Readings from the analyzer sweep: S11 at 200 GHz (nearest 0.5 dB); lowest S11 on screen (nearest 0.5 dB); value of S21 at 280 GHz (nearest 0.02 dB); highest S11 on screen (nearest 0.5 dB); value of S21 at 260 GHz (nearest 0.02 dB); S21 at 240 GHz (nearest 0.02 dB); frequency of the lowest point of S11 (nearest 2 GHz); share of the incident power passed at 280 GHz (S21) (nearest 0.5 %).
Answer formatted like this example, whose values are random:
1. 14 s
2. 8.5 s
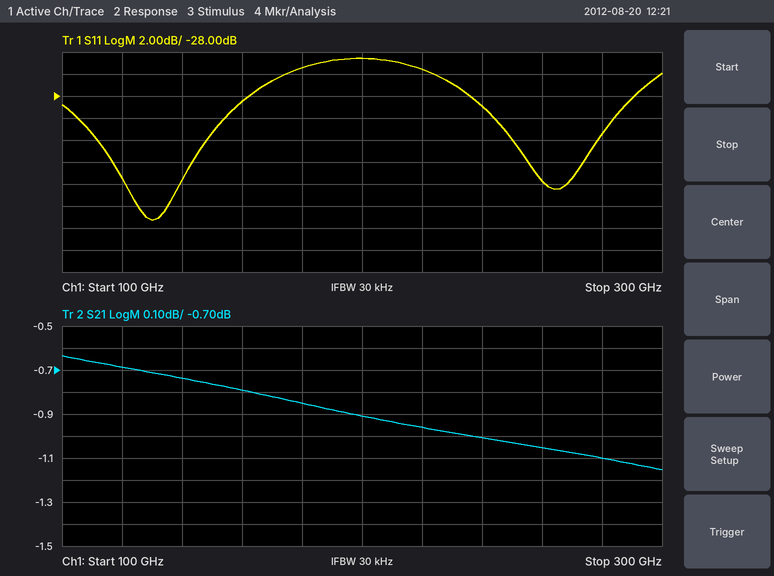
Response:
1. -24.5 dB
2. -39.5 dB
3. -1.10 dB
4. -24.5 dB
5. -1.06 dB
6. -1.00 dB
7. 130 GHz
8. 77.5 %
